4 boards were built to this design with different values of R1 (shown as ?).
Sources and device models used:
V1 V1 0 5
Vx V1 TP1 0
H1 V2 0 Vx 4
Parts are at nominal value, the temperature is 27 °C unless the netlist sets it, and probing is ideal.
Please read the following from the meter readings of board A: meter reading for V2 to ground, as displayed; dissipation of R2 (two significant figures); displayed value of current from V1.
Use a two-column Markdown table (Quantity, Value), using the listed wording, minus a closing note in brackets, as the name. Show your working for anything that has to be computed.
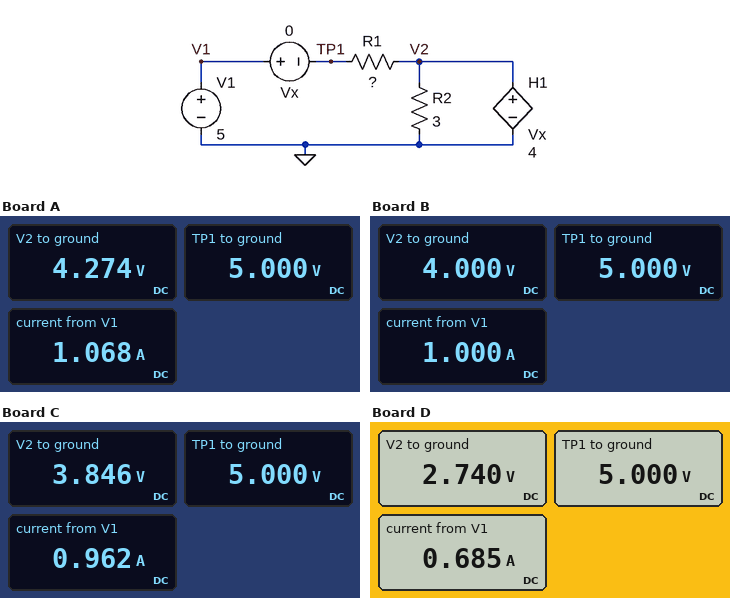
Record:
| Quantity | Value |
|---|---|
| meter reading for V2 to ground, as displayed | 4.274 V |
| dissipation of R2 | (4.274 V)^2 / 3 Ω = 6.1 W |
| displayed value of current from V1 | 1.068 A |
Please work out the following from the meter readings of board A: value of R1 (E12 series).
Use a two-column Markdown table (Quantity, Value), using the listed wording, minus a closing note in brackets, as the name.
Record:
| Quantity | Value |
|---|---|
| value of R1 | 0.68 Ω |
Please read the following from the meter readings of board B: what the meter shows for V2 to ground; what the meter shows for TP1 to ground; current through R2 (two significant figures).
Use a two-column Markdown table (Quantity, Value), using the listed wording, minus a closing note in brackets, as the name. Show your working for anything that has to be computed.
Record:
| Quantity | Value |
|---|---|
| what the meter shows for V2 to ground | 4.000 V |
| what the meter shows for TP1 to ground | 5.000 V |
| current through R2 | (4 V) / 3 Ω = 1.3 A |
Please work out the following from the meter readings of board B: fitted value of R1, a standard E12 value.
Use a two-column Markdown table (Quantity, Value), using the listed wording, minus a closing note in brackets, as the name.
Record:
| Quantity | Value |
|---|---|
| fitted value of R1, a standard E12 value | 1 Ω |
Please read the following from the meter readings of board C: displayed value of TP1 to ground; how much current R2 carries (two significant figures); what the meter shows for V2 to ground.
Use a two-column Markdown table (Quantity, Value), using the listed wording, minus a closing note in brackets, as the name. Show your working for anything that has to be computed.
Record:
| Quantity | Value |
|---|---|
| displayed value of TP1 to ground | 5.000 V |
| how much current R2 carries | (3.846 V) / 3 Ω = 1.3 A |
| what the meter shows for V2 to ground | 3.846 V |
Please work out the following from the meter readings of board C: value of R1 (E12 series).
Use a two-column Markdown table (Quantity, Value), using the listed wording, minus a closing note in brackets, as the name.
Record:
| Quantity | Value |
|---|---|
| value of R1 | 1.2 Ω |
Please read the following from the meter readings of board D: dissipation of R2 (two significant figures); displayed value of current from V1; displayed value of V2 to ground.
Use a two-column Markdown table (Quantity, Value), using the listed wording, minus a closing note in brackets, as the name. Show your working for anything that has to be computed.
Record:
| Quantity | Value |
|---|---|
| dissipation of R2 | (2.74 V)^2 / 3 Ω = 2.5 W |
| displayed value of current from V1 | 0.685 A |
| displayed value of V2 to ground | 2.740 V |
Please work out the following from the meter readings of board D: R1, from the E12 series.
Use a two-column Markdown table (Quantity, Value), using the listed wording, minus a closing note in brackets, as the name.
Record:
| Quantity | Value |
|---|---|
| R1, from the E12 series | 3.3 Ω |
